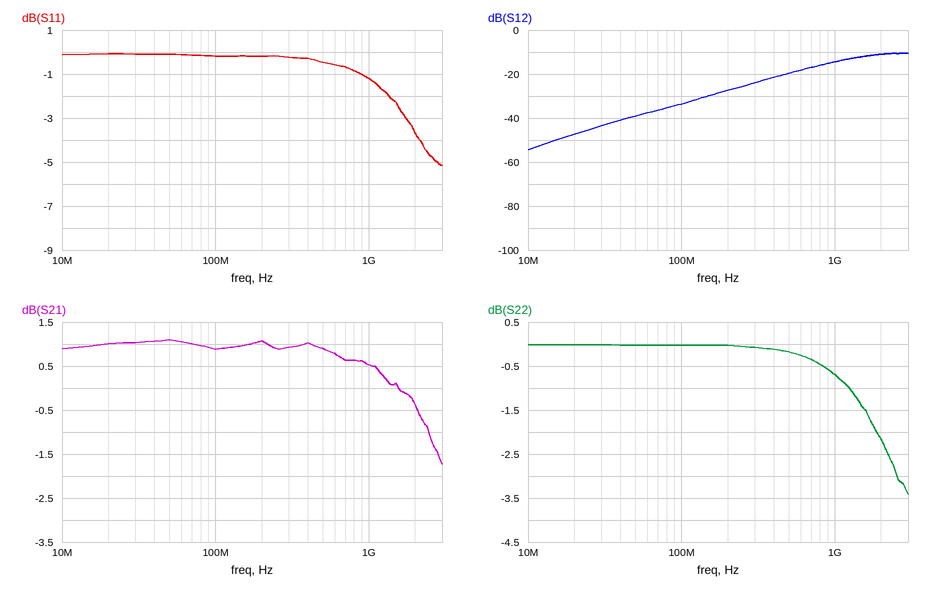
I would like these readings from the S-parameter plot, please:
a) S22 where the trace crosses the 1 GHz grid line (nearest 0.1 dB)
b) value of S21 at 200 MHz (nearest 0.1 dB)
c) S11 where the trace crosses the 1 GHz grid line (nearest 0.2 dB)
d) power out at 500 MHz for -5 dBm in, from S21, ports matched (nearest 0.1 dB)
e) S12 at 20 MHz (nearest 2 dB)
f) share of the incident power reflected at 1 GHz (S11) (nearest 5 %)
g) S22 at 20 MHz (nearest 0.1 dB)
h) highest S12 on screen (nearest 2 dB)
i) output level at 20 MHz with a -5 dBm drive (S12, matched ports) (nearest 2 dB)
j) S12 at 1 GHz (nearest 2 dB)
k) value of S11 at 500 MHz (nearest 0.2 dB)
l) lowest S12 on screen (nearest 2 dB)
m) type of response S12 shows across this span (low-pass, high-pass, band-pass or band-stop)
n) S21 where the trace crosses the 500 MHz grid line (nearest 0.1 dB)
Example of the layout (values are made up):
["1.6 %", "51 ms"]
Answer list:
["-0.7 dB", "1.1 dB", "-1.2 dB", "-4.1 dBm", "-48 dB", "75 %", "0.0 dB", "-10 dB", "-52 dBm", "-14 dB", "-0.4 dB", "-54 dB", "high-pass", "0.9 dB"]
